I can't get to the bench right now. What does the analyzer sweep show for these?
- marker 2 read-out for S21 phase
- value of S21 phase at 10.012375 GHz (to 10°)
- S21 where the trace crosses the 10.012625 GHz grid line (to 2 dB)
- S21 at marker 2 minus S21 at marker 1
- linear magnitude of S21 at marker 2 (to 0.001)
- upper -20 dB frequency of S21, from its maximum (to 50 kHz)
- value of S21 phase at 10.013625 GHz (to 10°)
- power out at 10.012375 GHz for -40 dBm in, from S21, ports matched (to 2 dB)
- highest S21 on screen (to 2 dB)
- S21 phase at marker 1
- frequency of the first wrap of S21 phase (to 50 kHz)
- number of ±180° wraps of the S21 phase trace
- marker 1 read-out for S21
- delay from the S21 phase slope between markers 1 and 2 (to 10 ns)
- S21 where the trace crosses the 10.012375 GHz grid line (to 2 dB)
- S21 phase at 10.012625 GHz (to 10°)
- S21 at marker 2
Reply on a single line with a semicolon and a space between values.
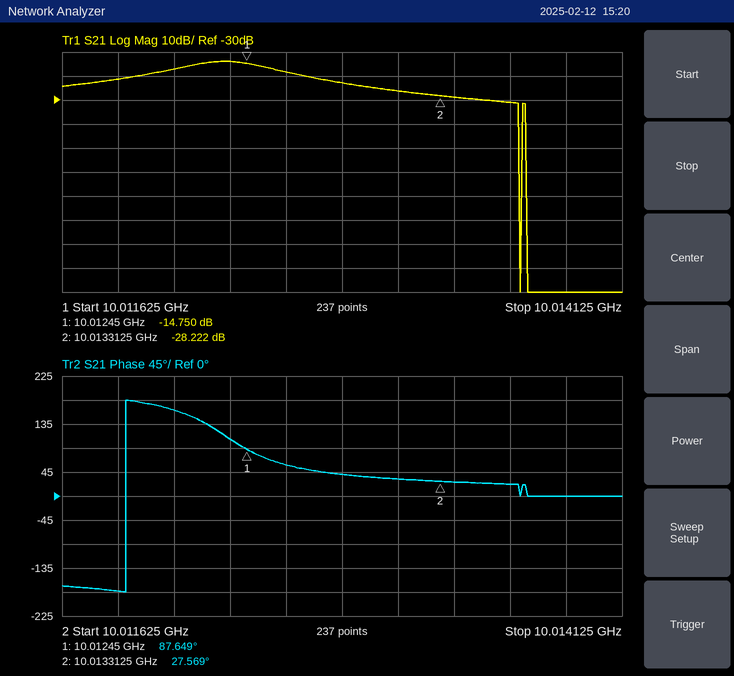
27.569°; 110°; -18 dB; -13.472 dB; 0.039; 10.01365 GHz; 20°; -54 dBm; -14 dB; 87.649°; 10.01190 GHz; 1; -14.750 dB; 190 ns; -14 dB; 60°; -28.222 dB
